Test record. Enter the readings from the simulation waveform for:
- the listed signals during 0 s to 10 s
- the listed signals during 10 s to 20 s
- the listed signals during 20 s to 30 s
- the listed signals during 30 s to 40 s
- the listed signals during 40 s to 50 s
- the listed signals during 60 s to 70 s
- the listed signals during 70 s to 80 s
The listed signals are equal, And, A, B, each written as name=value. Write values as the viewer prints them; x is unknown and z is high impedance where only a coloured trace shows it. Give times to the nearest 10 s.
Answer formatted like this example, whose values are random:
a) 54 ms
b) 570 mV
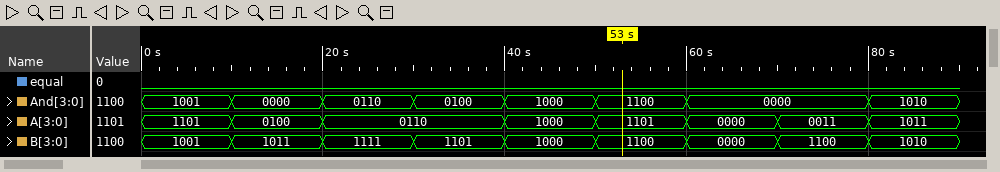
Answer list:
a) equal=0, And=1001, A=1101, B=1001
b) equal=0, And=0000, A=0100, B=1011
c) equal=0, And=0110, A=0110, B=1111
d) equal=0, And=0100, A=0110, B=1101
e) equal=0, And=1000, A=1000, B=1000
f) equal=0, And=0000, A=0000, B=0000
g) equal=0, And=0000, A=0011, B=1100
